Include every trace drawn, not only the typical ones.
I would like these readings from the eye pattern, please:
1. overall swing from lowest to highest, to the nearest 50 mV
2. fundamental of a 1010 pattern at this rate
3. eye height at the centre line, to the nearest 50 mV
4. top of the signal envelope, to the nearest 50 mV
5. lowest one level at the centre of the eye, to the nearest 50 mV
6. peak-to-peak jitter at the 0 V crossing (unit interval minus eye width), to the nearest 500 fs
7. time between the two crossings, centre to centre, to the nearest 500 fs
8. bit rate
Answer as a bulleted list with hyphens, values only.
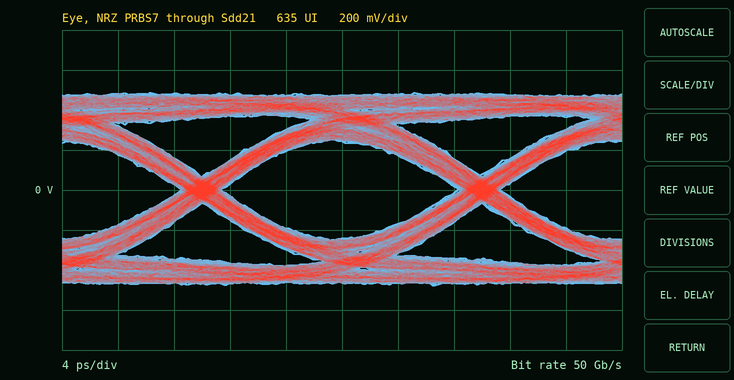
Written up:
- 950 mV
- 25 GHz
- 500 mV
- 500 mV
- 250 mV
- 3.0 ps
- 20.0 ps
- 50 Gb/s
